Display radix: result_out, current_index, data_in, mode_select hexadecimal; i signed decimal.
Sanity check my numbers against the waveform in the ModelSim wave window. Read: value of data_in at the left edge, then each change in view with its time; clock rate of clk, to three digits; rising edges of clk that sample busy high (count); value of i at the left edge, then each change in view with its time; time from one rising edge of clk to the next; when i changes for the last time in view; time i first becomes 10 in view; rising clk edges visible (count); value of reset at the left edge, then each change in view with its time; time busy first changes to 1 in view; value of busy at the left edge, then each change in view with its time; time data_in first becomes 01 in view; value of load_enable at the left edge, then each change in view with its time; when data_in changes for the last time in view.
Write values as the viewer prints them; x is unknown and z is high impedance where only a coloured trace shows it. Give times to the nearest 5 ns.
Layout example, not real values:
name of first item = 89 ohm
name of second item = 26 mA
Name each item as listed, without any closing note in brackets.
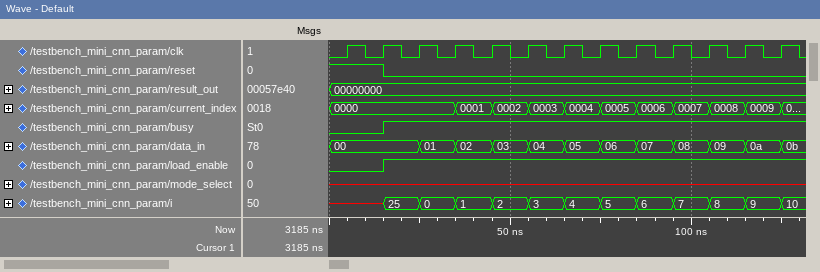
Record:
value of data_in at the left edge, then each change in view with its time = 00, 01 at 25 ns, 02 at 35 ns, 03 at 45 ns, 04 at 55 ns, 05 at 65 ns, 06 at 75 ns, 07 at 85 ns, 08 at 95 ns, 09 at 105 ns, 0a at 115 ns, 0b at 125 ns
clock rate of clk, to three digits = 100 MHz
rising edges of clk that sample busy high = 11
value of i at the left edge, then each change in view with its time = x, 25 at 15 ns, 0 at 25 ns, 1 at 35 ns, 2 at 45 ns, 3 at 55 ns, 4 at 65 ns, 5 at 75 ns, 6 at 85 ns, 7 at 95 ns, 8 at 105 ns, 9 at 115 ns, 10 at 125 ns
time from one rising edge of clk to the next = 10 ns
when i changes for the last time in view = 125 ns
time i first becomes 10 in view = 125 ns
rising clk edges visible = 13
value of reset at the left edge, then each change in view with its time = 1, 0 at 15 ns
time busy first changes to 1 in view = 15 ns
value of busy at the left edge, then each change in view with its time = 0, 1 at 15 ns
time data_in first becomes 01 in view = 25 ns
value of load_enable at the left edge, then each change in view with its time = 0, 1 at 15 ns
when data_in changes for the last time in view = 125 ns
